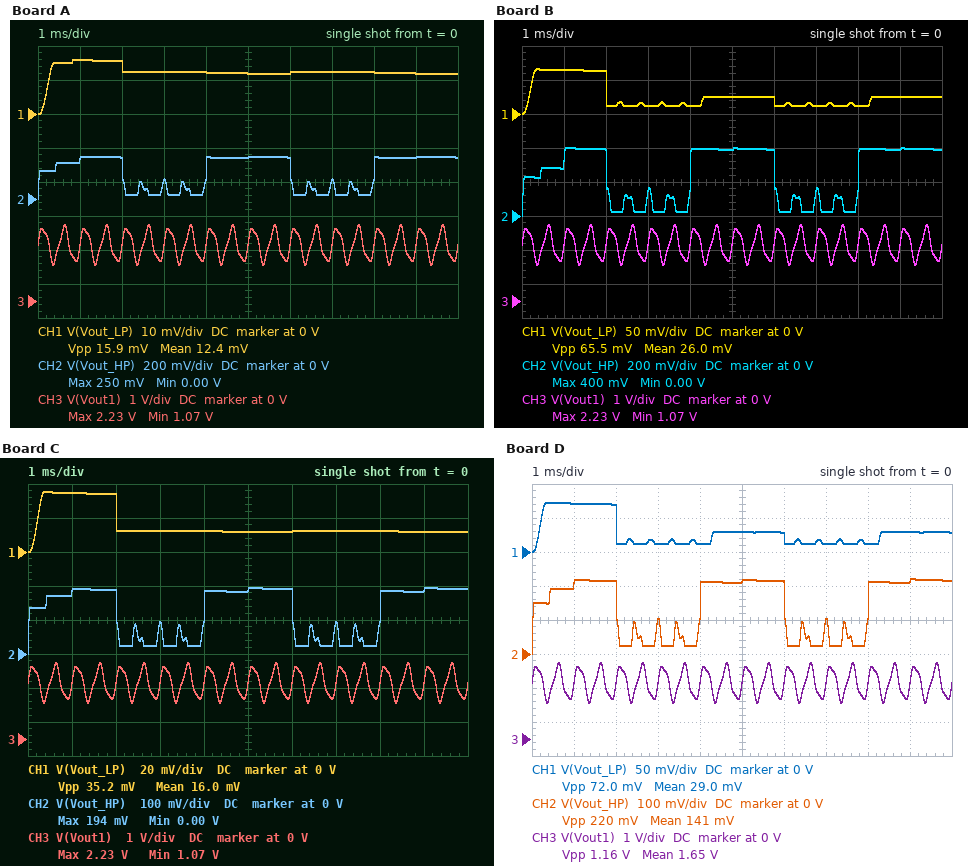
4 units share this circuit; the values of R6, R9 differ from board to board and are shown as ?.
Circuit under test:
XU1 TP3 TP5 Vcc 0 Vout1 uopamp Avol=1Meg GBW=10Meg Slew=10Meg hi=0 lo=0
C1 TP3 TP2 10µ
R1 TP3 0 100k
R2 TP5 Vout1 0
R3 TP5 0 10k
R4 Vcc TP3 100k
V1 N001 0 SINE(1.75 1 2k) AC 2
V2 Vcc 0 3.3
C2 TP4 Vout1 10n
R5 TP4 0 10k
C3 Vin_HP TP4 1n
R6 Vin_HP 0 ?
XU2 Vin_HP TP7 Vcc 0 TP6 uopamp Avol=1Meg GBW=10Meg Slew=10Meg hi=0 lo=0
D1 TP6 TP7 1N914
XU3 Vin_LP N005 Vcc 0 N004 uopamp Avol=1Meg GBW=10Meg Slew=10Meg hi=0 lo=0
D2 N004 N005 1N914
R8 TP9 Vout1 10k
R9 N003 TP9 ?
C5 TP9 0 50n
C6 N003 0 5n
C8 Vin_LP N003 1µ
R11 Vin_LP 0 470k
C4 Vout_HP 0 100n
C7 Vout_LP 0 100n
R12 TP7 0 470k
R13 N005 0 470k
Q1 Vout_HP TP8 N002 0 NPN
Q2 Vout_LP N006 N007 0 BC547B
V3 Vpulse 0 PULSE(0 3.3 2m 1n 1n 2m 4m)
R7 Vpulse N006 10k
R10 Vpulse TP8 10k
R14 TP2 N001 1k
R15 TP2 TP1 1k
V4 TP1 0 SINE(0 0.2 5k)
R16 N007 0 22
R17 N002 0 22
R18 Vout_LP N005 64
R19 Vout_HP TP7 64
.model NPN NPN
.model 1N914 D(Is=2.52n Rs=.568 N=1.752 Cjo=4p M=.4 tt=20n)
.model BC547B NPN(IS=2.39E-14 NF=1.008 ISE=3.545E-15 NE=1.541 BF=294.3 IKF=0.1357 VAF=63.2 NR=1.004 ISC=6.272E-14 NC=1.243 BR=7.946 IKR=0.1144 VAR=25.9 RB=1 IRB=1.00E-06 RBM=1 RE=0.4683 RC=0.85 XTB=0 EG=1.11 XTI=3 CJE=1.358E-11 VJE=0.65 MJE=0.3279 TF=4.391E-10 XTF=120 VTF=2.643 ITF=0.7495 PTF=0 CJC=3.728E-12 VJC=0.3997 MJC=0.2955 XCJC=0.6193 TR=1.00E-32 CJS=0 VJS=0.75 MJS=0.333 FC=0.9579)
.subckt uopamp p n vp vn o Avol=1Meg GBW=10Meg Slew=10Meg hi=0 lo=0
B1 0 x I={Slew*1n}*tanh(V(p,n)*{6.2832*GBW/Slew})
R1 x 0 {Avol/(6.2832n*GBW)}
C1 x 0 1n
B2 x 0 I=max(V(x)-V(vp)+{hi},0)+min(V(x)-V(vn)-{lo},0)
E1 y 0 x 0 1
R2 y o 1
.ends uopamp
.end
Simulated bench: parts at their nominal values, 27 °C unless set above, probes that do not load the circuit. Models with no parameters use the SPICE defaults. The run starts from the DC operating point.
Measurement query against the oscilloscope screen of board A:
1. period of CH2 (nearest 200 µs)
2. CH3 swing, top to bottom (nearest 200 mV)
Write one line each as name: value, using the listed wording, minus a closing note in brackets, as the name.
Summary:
period of CH2: 4.0 ms
CH3 swing, top to bottom: 1.2 V
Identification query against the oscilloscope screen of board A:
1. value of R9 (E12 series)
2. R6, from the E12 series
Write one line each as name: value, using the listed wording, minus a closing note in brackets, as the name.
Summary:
value of R9: 330 kΩ
R6, from the E12 series: 47 kΩ
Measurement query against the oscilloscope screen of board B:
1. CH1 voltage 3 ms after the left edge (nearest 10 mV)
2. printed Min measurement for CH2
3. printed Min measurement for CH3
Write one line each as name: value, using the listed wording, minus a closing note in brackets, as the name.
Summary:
CH1 voltage 3 ms after the left edge: 10 mV
printed Min measurement for CH2: 0.00 V
printed Min measurement for CH3: 1.07 V
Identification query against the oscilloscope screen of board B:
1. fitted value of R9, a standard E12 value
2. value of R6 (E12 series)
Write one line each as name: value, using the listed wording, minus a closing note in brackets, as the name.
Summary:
fitted value of R9, a standard E12 value: 47 kΩ
value of R6: 120 kΩ
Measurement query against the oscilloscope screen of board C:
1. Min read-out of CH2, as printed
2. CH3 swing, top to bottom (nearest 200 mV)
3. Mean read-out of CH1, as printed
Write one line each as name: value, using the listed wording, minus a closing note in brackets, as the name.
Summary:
Min read-out of CH2, as printed: 0.00 V
CH3 swing, top to bottom: 1.2 V
Mean read-out of CH1, as printed: 16.0 mV
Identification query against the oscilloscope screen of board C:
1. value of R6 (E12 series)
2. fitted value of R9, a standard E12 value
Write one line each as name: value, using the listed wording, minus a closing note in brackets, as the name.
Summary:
value of R6: 33 kΩ
fitted value of R9, a standard E12 value: 120 kΩ
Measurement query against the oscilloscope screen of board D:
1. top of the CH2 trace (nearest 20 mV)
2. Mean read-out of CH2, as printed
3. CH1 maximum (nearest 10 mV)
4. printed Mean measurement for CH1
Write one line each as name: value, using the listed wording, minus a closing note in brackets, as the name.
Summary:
top of the CH2 trace: 220 mV
Mean read-out of CH2, as printed: 141 mV
CH1 maximum: 70 mV
printed Mean measurement for CH1: 29.0 mV
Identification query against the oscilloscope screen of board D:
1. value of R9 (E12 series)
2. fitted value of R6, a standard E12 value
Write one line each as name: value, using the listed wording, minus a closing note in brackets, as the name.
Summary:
value of R9: 39 kΩ
fitted value of R6, a standard E12 value: 39 kΩ
